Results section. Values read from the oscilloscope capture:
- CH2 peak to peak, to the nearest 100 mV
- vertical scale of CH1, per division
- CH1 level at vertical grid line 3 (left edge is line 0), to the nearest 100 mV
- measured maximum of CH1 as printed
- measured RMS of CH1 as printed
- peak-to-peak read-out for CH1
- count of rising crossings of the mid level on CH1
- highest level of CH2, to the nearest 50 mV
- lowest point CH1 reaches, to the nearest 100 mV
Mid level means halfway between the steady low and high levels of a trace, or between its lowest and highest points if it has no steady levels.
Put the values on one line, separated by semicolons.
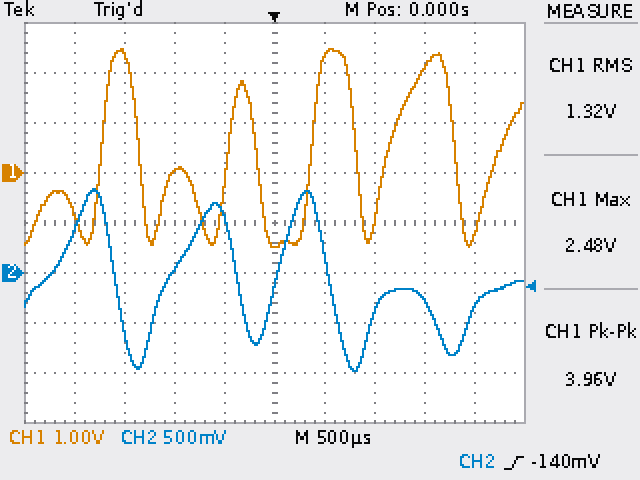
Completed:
1.80 V; 1 V; 0.0 V; 2.48 V; 1.32 V; 3.96 V; 5; 850 mV; -1.5 V
